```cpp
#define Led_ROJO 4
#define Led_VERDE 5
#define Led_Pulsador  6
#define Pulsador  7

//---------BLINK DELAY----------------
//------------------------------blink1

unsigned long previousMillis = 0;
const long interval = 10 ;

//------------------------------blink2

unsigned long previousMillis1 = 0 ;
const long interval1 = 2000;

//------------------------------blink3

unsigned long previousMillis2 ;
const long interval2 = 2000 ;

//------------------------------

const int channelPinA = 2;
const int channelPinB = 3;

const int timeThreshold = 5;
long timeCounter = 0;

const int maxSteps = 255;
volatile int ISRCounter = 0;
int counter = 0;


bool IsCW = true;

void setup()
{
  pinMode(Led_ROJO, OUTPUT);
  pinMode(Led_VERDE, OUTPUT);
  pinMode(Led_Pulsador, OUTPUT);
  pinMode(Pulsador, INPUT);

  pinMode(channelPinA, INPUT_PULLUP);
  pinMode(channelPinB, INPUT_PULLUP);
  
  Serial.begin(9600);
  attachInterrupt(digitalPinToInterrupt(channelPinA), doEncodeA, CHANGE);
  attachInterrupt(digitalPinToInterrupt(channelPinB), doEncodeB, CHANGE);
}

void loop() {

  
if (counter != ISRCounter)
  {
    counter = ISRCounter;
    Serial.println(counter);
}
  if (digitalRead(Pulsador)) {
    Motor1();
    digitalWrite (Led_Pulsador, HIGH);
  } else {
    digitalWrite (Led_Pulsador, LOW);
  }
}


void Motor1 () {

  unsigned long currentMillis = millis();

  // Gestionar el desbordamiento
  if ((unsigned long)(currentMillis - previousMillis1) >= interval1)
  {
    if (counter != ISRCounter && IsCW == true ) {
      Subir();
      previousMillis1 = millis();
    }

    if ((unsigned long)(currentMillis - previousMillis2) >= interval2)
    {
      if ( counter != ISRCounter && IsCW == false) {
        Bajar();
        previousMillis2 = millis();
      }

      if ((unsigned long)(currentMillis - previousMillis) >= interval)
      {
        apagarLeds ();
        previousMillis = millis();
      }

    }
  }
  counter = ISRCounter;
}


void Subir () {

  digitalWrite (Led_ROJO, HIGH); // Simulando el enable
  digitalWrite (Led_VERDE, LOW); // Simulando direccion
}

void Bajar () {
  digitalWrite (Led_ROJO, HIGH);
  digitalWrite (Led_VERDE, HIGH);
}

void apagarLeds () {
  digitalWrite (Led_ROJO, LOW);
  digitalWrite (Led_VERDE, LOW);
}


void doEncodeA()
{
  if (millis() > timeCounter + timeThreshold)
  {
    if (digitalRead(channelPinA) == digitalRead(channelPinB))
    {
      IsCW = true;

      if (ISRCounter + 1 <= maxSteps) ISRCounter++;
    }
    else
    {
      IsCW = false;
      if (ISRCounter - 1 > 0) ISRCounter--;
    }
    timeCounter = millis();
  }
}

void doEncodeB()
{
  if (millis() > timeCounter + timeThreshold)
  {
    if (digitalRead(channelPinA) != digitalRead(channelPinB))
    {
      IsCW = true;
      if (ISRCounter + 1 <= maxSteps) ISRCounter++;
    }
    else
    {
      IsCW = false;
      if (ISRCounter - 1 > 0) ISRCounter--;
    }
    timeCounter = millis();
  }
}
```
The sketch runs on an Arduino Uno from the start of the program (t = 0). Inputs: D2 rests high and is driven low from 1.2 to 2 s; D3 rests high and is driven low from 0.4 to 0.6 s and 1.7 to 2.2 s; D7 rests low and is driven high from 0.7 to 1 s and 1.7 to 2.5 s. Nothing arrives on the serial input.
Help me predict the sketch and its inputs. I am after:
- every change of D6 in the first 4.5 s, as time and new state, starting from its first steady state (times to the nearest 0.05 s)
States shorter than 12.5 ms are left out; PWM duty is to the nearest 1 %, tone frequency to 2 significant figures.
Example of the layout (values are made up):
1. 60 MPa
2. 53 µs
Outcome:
1. 0 s low; 0.7 s high; 1 s low; 1.7 s high; 2.5 s low
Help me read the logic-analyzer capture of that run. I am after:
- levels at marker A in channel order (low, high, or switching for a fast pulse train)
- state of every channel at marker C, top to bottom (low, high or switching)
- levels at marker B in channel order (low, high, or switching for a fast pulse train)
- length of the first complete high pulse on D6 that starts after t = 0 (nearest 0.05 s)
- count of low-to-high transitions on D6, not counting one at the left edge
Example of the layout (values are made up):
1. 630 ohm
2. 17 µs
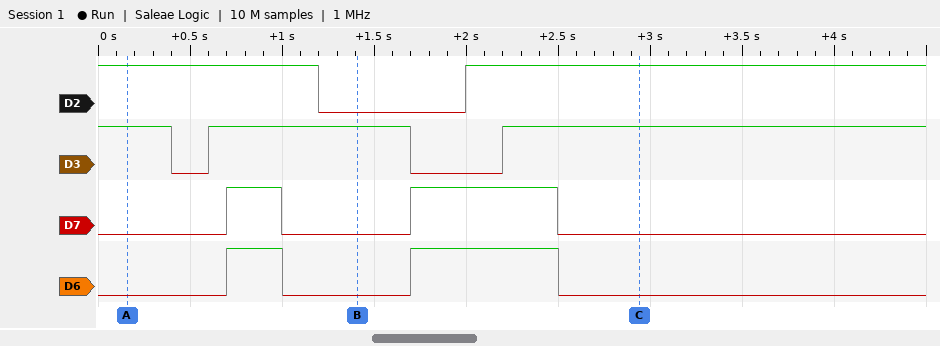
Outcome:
1. D2 high, D3 high, D7 low, D6 low
2. D2 high, D3 high, D7 low, D6 low
3. D2 low, D3 high, D7 low, D6 low
4. 0.30 s
5. 2
